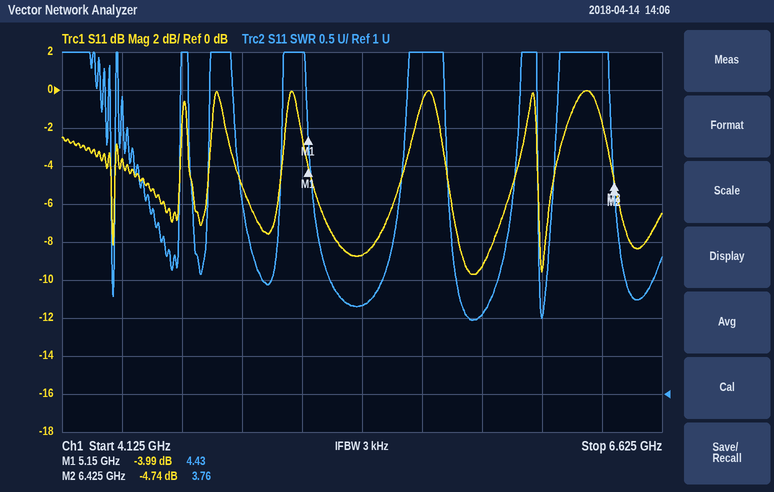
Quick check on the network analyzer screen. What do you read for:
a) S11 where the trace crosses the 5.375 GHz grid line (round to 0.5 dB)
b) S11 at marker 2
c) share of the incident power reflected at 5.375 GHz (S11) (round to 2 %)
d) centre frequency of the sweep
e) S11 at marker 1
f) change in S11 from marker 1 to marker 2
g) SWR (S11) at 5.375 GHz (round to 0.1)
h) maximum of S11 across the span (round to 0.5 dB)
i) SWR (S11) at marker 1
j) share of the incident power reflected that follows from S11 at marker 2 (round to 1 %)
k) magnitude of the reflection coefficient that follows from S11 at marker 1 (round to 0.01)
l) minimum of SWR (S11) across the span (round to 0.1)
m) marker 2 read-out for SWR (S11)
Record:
-8.5 dB
-4.74 dB
14 %
5.375 GHz
-3.99 dB
-0.75 dB
2.2
0.0 dB
4.43
34 %
0.63
2.0
3.76
